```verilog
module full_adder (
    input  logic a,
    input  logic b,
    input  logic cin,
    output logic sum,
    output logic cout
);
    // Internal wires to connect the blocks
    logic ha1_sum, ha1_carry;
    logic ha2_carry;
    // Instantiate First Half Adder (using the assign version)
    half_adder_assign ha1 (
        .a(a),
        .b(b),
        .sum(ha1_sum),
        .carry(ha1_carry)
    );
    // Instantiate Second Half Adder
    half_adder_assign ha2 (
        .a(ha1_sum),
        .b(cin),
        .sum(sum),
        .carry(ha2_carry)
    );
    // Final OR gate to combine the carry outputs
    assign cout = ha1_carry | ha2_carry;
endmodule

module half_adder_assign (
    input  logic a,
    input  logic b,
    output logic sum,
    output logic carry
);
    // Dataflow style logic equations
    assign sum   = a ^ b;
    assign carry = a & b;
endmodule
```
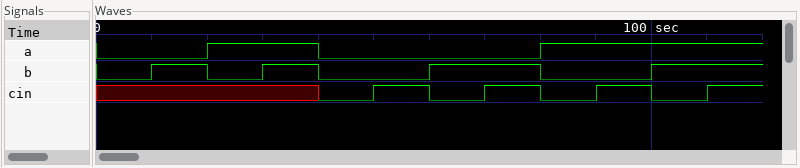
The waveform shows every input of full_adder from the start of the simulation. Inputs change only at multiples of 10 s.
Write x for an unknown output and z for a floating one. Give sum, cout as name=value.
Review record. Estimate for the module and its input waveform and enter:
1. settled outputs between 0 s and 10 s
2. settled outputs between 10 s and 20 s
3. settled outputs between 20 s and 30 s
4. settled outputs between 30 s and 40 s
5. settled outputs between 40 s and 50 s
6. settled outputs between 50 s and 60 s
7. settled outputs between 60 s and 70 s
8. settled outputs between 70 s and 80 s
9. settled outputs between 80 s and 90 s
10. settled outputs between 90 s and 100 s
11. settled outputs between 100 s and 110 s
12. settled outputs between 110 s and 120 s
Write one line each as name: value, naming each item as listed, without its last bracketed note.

settled outputs between 0 s and 10 s: sum=x, cout=0
settled outputs between 10 s and 20 s: sum=x, cout=x
settled outputs between 20 s and 30 s: sum=x, cout=x
settled outputs between 30 s and 40 s: sum=x, cout=1
settled outputs between 40 s and 50 s: sum=0, cout=0
settled outputs between 50 s and 60 s: sum=1, cout=0
settled outputs between 60 s and 70 s: sum=1, cout=0
settled outputs between 70 s and 80 s: sum=0, cout=1
settled outputs between 80 s and 90 s: sum=1, cout=0
settled outputs between 90 s and 100 s: sum=0, cout=1
settled outputs between 100 s and 110 s: sum=0, cout=1
settled outputs between 110 s and 120 s: sum=1, cout=1
